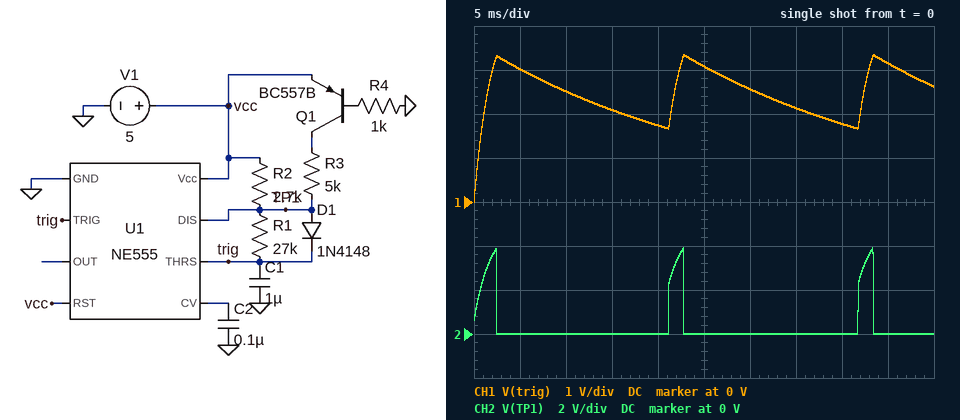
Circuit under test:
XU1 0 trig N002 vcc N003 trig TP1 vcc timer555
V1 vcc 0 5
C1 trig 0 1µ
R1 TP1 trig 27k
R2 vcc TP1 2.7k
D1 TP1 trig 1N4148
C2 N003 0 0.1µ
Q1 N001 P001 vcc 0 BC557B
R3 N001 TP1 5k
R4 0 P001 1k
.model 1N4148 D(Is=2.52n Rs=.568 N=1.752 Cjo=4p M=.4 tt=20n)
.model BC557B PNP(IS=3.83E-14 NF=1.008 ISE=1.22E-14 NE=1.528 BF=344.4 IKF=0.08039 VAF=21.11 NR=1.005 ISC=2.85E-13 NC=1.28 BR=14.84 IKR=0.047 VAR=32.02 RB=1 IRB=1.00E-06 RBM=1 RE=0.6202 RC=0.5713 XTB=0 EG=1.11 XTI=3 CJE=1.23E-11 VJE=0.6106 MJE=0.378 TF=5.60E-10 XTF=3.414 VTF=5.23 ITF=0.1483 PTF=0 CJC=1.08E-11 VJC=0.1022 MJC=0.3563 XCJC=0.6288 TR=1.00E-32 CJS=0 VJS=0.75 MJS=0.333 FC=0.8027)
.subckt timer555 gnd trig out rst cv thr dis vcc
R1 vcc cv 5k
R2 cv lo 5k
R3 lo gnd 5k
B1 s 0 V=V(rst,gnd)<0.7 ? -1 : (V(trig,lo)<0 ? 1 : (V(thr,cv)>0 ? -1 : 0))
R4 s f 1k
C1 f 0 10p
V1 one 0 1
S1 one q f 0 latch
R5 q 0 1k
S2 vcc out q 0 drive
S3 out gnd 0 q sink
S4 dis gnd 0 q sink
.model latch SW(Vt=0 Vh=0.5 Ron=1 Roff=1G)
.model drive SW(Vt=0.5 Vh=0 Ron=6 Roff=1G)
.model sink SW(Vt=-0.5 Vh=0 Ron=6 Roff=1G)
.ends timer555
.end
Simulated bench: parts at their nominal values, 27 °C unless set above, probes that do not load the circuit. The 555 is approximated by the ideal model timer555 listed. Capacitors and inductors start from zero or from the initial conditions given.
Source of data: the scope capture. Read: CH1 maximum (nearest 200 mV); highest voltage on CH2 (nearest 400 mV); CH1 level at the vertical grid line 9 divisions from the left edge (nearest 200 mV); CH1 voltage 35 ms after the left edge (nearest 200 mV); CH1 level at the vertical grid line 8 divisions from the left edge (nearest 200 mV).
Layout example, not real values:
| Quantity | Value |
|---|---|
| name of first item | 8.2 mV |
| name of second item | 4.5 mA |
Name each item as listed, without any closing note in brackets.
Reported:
| Quantity | Value |
|---|---|
| CH1 maximum | 3.4 V |
| highest voltage on CH2 | 4.0 V |
| CH1 level at the vertical grid line 9 divisions from the left edge | 3.2 V |
| CH1 voltage 35 ms after the left edge | 2.2 V |
| CH1 level at the vertical grid line 8 divisions from the left edge | 1.8 V |
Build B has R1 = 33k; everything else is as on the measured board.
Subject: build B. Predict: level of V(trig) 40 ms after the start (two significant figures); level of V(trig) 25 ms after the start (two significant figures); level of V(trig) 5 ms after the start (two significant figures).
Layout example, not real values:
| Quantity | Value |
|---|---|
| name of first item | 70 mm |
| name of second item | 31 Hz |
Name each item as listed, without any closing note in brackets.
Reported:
| Quantity | Value |
|---|---|
| level of V(trig) 40 ms after the start | 2.3 V |
| level of V(trig) 25 ms after the start | 1.7 V |
| level of V(trig) 5 ms after the start | 3.1 V |
